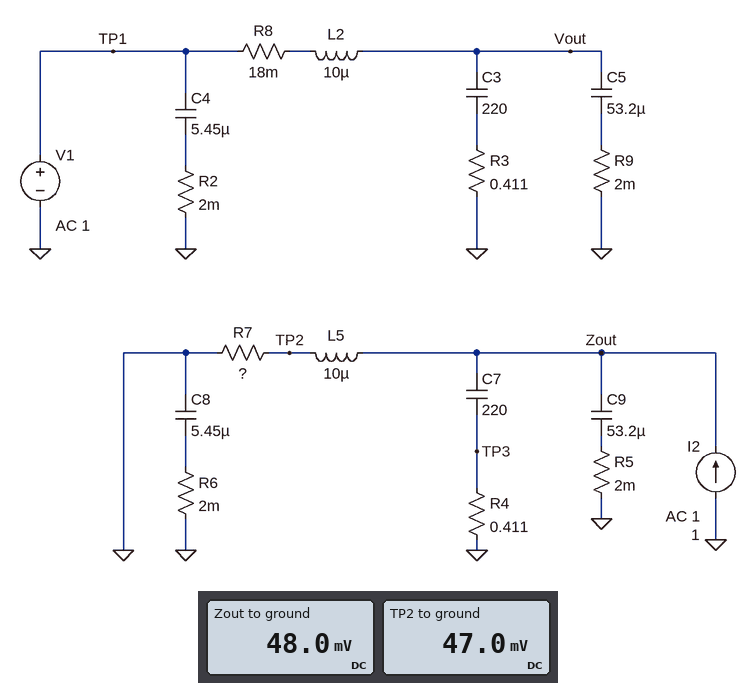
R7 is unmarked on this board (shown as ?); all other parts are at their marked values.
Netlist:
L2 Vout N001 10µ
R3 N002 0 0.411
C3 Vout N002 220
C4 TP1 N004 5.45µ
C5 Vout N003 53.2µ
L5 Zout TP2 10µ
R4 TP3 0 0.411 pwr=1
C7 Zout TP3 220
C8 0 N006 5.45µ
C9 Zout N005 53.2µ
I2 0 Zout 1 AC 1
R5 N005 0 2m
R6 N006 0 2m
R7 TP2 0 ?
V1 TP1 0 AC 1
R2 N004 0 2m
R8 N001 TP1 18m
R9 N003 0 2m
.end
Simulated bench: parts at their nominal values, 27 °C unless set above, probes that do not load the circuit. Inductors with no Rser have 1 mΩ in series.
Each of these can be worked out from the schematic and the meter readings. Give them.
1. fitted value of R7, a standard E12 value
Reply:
0.047 Ω
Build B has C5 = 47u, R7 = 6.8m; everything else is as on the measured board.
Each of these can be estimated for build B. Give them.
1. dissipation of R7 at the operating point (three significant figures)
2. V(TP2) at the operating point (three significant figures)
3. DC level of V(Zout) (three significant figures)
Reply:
6.80 mW
6.80 mV
7.80 mV
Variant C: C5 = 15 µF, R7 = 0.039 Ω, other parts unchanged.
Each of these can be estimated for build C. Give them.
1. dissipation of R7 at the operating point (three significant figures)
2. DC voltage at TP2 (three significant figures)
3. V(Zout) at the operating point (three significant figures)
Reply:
39.0 mW
39.0 mV
40.0 mV
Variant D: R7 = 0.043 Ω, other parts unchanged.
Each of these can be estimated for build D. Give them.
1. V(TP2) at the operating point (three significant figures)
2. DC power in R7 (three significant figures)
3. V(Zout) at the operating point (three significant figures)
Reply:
43.0 mV
43.0 mW
44.0 mV
